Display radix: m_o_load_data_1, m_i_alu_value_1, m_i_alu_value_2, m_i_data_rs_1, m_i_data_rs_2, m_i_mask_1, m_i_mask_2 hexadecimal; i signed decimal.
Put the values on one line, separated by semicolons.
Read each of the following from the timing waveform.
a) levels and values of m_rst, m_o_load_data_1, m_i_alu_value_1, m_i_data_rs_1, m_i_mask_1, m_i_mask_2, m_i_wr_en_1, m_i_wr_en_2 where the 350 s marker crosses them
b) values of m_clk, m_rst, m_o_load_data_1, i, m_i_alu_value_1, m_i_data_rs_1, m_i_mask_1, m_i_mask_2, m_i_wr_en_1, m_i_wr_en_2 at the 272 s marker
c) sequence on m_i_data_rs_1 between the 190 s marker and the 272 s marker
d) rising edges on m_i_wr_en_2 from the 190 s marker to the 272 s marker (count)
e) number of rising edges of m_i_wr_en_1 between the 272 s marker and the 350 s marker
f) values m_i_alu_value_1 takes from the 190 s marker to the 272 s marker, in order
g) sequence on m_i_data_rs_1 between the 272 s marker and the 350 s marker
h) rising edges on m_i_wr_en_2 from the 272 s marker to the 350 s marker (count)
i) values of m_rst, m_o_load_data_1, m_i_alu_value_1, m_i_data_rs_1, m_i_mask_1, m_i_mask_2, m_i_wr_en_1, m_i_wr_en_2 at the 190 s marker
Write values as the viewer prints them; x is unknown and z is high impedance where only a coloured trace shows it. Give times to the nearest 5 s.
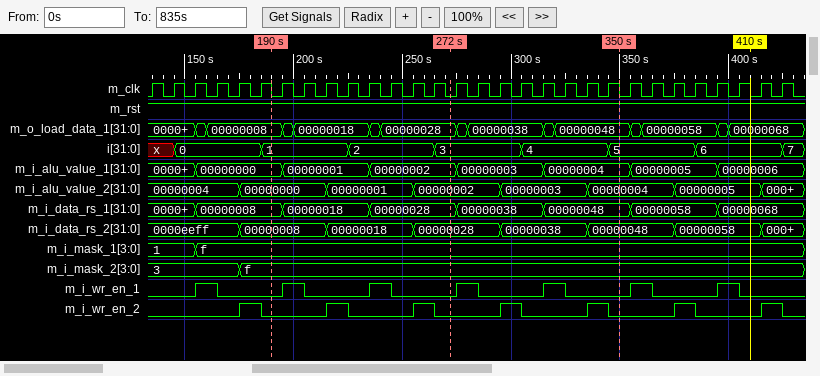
m_rst=1, m_o_load_data_1=00000048, m_i_alu_value_1=00000004, m_i_data_rs_1=00000048, m_i_mask_1=f, m_i_mask_2=f, m_i_wr_en_1=0, m_i_wr_en_2=0; m_clk=0, m_rst=1, m_o_load_data_1=00000028, i=3, m_i_alu_value_1=00000002, m_i_data_rs_1=00000028, m_i_mask_1=f, m_i_mask_2=f, m_i_wr_en_1=0, m_i_wr_en_2=0; 00000008, 00000018, 00000028; 2; 2; 00000000, 00000001, 00000002; 00000028, 00000038, 00000048; 2; m_rst=1, m_o_load_data_1=00000008, m_i_alu_value_1=00000000, m_i_data_rs_1=00000008, m_i_mask_1=f, m_i_mask_2=f, m_i_wr_en_1=0, m_i_wr_en_2=0
